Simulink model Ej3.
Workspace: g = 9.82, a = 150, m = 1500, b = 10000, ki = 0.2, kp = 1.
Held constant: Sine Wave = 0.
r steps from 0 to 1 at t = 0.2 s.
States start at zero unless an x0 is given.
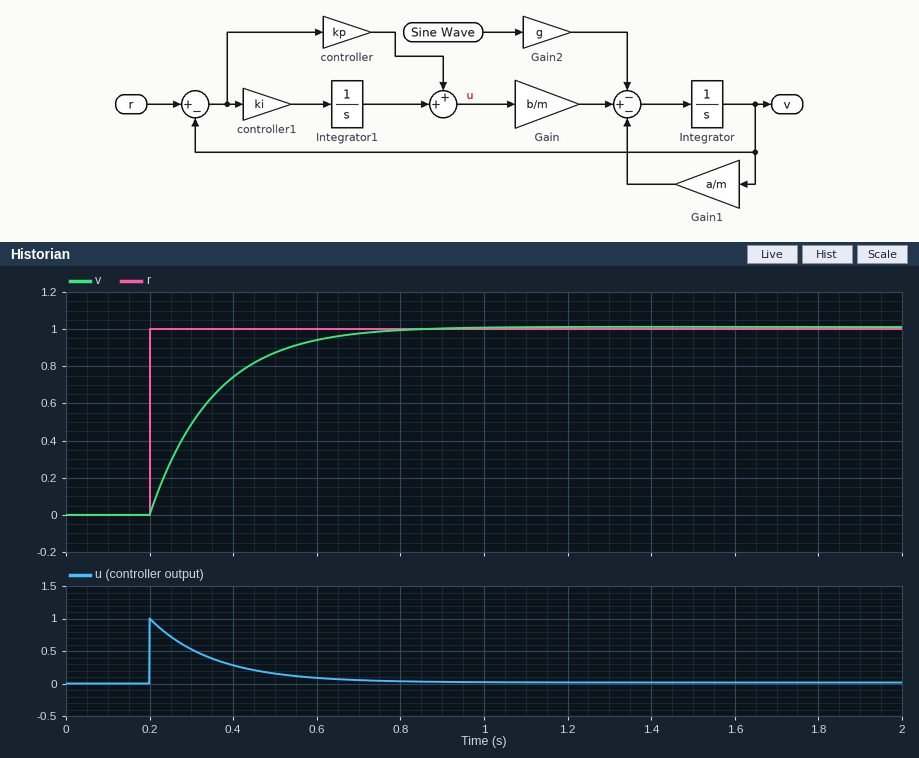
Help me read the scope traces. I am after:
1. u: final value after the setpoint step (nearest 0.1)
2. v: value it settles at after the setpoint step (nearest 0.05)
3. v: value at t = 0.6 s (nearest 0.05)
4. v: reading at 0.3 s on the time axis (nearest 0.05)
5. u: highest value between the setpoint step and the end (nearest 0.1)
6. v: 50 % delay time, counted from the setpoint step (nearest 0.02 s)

0.0
1.00
0.95
0.50
1.0
0.10 s
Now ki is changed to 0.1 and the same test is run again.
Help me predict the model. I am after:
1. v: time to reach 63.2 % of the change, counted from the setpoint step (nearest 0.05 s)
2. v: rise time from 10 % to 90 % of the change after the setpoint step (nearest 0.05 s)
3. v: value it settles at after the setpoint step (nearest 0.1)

0.15 s
0.35 s
1.0
